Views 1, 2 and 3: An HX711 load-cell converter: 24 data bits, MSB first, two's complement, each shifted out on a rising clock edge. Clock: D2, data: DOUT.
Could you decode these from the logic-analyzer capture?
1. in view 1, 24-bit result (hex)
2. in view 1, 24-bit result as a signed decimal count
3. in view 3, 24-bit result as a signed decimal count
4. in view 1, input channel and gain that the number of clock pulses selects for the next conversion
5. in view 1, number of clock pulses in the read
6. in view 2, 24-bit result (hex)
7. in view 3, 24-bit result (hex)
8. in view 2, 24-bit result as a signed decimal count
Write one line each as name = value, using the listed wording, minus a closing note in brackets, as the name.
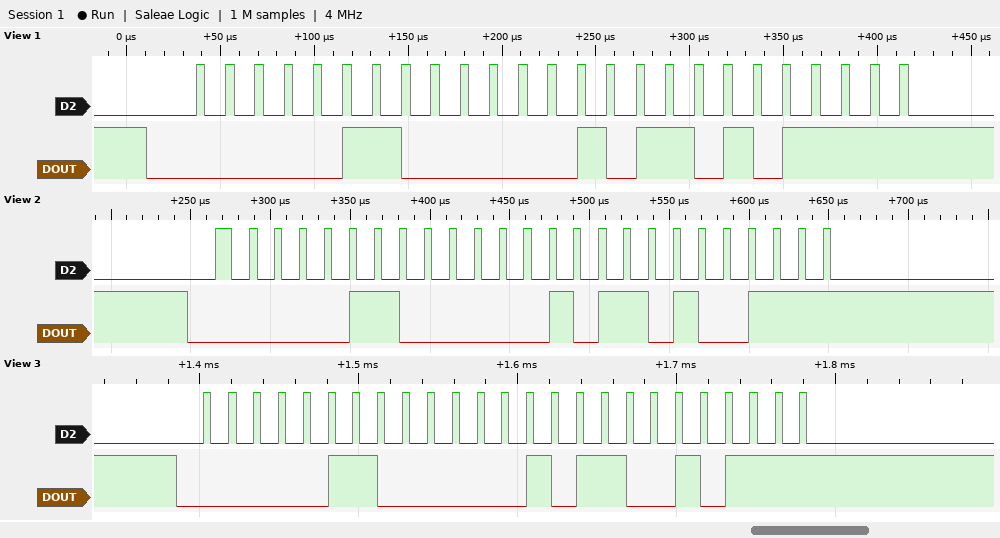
in view 1, 24-bit result = 0x0605AF
in view 1, 24-bit result as a signed decimal count = 394671
in view 3, 24-bit result as a signed decimal count = 394647
in view 1, input channel and gain that the number of clock pulses selects for the next conversion = channel A, gain 128
in view 1, number of clock pulses in the read = 25
in view 2, 24-bit result = 0x0605A7
in view 3, 24-bit result = 0x060597
in view 2, 24-bit result as a signed decimal count = 394663
